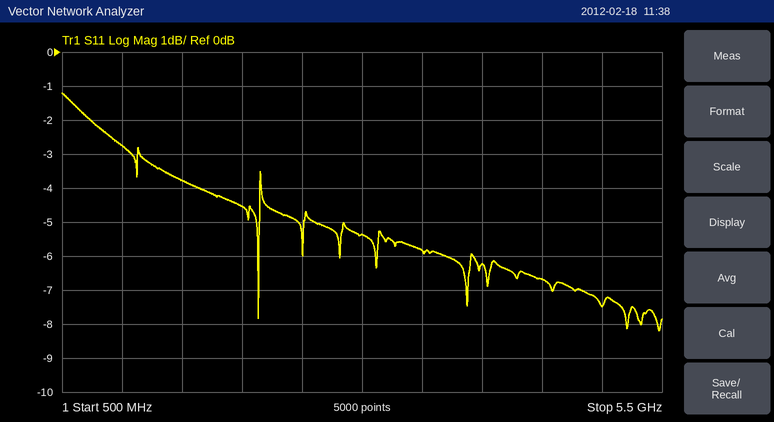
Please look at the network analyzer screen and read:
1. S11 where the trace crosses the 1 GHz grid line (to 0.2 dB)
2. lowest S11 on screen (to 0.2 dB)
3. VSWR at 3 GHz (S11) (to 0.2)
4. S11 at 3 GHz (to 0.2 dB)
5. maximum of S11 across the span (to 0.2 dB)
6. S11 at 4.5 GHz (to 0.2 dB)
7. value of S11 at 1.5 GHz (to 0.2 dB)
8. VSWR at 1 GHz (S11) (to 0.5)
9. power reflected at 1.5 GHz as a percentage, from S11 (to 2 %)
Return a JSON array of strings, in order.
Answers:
["-2.8 dB", "-8.2 dB", "3.4", "-5.4 dB", "-1.2 dB", "-6.6 dB", "-3.8 dB", "6.5", "42 %"]
